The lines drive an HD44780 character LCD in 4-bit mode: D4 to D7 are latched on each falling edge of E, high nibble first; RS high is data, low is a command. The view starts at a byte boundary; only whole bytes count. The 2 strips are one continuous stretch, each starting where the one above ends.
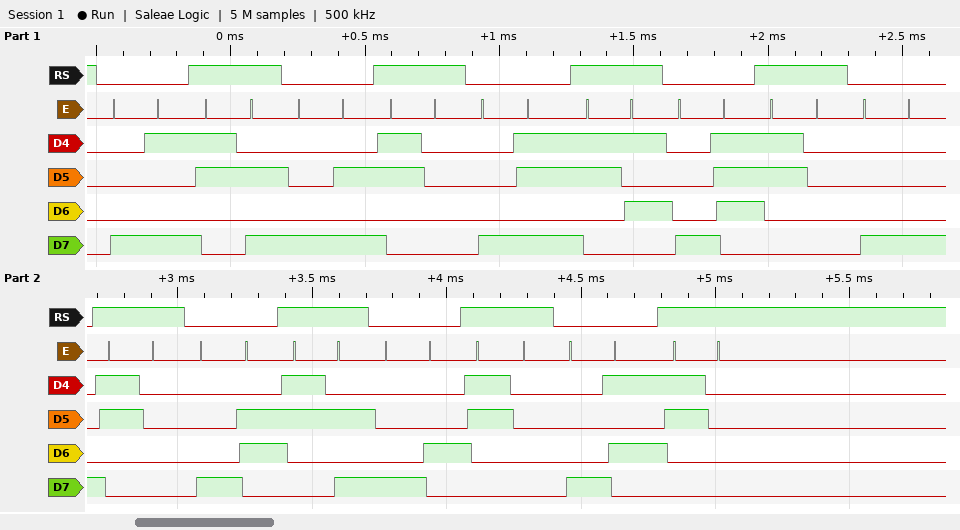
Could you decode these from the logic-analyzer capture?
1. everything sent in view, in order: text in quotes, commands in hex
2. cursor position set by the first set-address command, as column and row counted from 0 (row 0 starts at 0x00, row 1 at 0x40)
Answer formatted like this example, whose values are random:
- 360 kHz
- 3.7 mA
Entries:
- 0x89 ":" 0x8A "0" 0x8B "5" 0x87 "0" 0x88 "0" 0x86 ":" 0x84 "0" 0x85 "0"
- column 9, row 0
